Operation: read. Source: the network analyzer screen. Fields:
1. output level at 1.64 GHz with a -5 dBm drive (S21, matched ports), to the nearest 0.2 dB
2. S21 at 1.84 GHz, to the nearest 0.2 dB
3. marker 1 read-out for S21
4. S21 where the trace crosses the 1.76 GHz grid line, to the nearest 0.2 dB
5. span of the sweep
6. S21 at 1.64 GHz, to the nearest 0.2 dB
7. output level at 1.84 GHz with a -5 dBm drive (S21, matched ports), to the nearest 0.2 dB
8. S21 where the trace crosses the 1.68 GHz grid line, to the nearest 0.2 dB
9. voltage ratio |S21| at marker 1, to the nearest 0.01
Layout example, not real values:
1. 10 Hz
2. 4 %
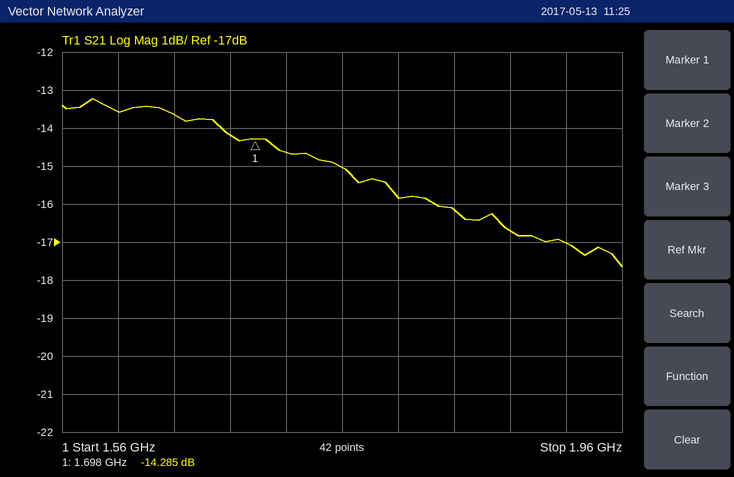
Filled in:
1. -18.6 dBm
2. -16.2 dB
3. -14.285 dB
4. -15.0 dB
5. 400 MHz
6. -13.6 dB
7. -21.2 dBm
8. -14.2 dB
9. 0.19
